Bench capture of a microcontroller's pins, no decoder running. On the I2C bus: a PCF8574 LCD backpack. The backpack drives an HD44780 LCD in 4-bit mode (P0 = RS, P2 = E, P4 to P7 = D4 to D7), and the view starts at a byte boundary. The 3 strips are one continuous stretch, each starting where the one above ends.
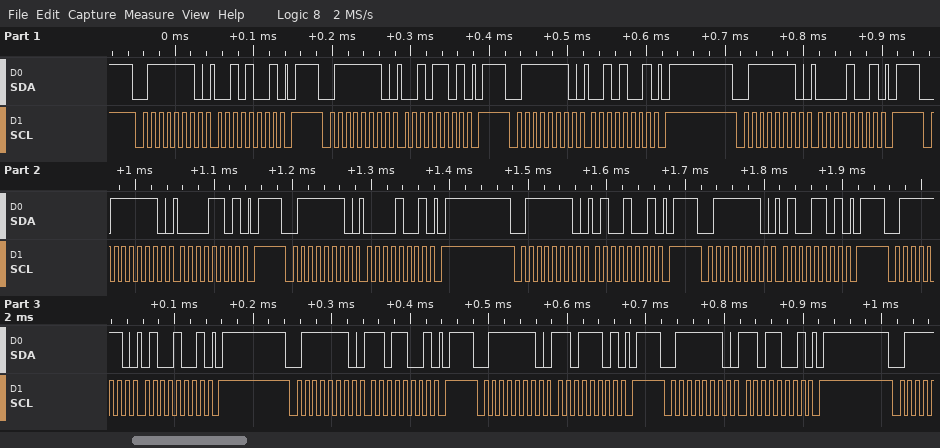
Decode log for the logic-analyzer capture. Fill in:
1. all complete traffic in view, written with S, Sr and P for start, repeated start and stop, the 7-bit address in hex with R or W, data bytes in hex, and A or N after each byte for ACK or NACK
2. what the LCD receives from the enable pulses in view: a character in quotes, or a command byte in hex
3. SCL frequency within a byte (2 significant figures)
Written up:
S 3FW A 29 A P S 3FW A 2D A P S 3FW A 29 A P S 3FW A 09 A P S 3FW A 0D A P S 3FW A 09 A P S 3FW A 49 A P S 3FW A 4D A P S 3FW A 49 A P S 3FW A D9 A P S 3FW A DD A P S 3FW A D9 A P
' ' 'M'
100 kHz
